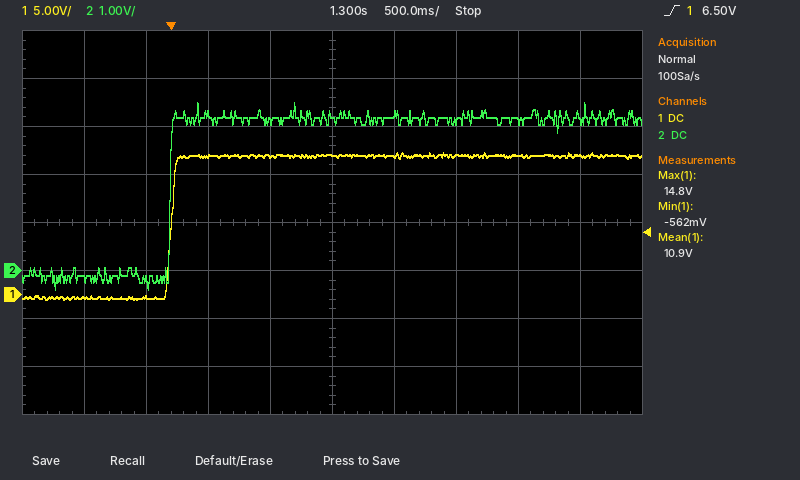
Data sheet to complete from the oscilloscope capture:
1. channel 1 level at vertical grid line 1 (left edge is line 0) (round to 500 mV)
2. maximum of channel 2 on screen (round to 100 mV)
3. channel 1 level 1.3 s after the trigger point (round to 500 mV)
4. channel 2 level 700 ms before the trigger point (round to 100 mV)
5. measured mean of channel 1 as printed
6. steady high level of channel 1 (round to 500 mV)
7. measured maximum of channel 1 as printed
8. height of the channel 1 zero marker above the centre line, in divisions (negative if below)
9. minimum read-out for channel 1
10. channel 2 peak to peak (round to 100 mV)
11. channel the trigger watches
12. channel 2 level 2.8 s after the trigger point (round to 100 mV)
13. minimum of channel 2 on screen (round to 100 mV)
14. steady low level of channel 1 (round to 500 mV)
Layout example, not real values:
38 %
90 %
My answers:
-500 mV
3.5 V
14.5 V
-200 mV
10.9 V
14.5 V
14.8 V
-1.5 div
-562 mV
3.9 V
channel 1
3.1 V
-400 mV
-500 mV
